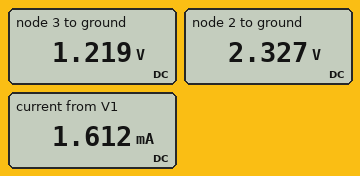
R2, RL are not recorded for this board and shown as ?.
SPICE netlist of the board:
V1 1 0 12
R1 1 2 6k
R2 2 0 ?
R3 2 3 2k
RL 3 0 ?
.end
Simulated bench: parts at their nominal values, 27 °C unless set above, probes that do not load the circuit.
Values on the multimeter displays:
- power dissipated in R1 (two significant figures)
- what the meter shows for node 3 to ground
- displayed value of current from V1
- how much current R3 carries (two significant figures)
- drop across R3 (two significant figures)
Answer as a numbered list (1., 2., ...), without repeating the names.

1. 16 mW
2. 1.219 V
3. 1.612 mA
4. 550 µA
5. 1.1 V
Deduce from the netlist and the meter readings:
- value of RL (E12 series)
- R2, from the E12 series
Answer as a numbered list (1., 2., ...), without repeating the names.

1. 2.2 kΩ
2. 2.2 kΩ
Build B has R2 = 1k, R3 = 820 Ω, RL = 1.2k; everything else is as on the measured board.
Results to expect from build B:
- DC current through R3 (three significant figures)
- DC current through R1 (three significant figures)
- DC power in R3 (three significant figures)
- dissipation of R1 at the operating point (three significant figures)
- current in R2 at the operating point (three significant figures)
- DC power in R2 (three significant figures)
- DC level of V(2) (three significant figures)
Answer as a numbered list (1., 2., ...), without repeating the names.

1. 596 µA
2. 1.80 mA
3. 291 µW
4. 19.4 mW
5. 1.20 mA
6. 1.45 mW
7. 1.20 V
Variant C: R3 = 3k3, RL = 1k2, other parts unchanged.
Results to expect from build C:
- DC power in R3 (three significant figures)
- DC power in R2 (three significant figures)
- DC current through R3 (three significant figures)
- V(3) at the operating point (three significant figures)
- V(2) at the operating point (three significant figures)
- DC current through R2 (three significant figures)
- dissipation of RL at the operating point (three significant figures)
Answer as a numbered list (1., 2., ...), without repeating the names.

1. 916 µW
2. 2.56 mW
3. 527 µA
4. 632 mV
5. 2.37 V
6. 1.08 mA
7. 333 µW
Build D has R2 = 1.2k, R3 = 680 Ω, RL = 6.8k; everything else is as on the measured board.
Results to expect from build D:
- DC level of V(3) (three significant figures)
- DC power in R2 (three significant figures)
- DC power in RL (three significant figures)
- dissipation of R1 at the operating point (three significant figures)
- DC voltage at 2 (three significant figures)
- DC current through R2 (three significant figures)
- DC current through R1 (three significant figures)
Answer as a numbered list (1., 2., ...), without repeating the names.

1. 1.60 V
2. 2.59 mW
3. 378 µW
4. 17.5 mW
5. 1.76 V
6. 1.47 mA
7. 1.71 mA
